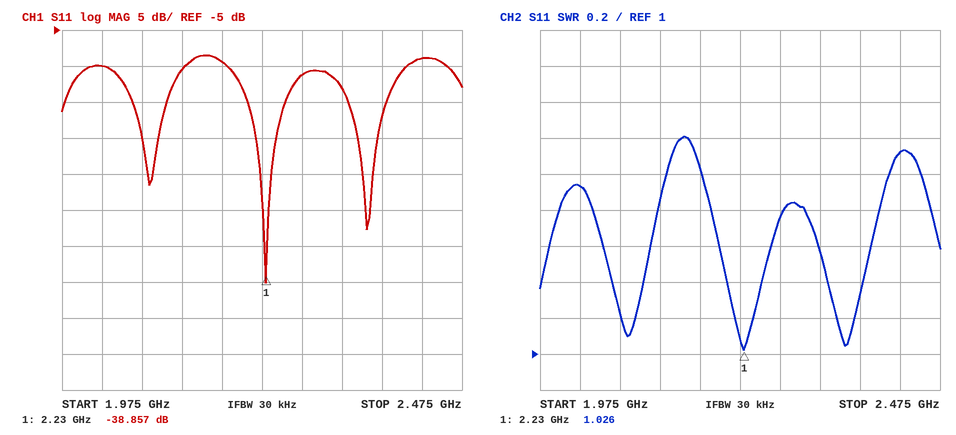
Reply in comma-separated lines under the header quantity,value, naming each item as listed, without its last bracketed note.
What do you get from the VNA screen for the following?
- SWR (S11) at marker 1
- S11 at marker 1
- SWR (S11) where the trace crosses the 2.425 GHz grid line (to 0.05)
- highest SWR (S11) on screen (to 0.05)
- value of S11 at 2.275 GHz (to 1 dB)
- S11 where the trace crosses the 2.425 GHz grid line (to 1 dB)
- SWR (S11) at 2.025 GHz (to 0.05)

quantity,value
SWR (S11) at marker 1,1.026
S11 at marker 1,-38.857 dB
SWR (S11) where the trace crosses the 2.425 GHz grid line,2.10
highest SWR (S11) on screen,2.20
value of S11 at 2.275 GHz,-11 dB
S11 where the trace crosses the 2.425 GHz grid line,-9 dB
SWR (S11) at 2.025 GHz,1.95
